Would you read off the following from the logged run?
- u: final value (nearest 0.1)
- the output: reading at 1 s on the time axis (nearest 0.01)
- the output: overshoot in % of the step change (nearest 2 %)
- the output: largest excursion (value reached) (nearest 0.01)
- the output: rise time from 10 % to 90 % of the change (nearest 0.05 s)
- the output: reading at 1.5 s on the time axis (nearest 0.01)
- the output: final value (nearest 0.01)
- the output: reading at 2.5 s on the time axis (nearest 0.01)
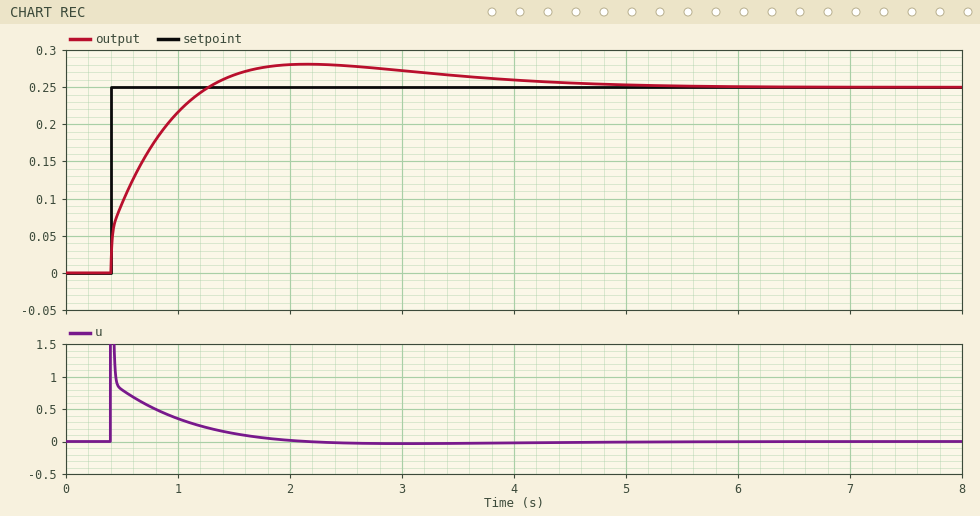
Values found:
0.0
0.22
12 %
0.28
0.65 s
0.27
0.25
0.28
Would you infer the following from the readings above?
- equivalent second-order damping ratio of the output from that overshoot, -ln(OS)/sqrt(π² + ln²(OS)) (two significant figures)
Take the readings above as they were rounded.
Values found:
0.56
